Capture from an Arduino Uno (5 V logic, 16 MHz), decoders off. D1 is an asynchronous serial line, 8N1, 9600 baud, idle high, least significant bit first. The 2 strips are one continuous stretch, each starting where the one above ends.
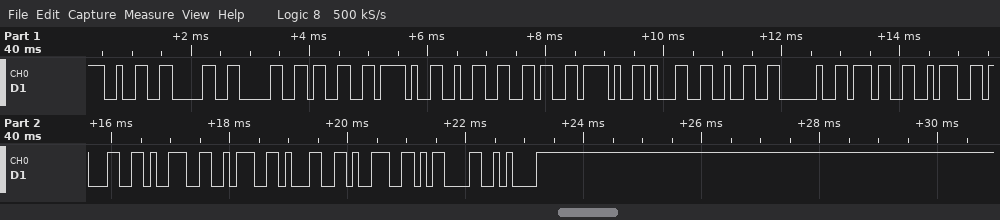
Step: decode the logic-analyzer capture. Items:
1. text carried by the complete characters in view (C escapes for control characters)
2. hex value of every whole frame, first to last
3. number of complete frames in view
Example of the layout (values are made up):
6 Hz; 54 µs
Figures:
"2003/26/12 7:19:19\r\n"; 0x32 0x30 0x30 0x33 0x2F 0x32 0x36 0x2F 0x31 0x32 0x20 0x37 0x3A 0x31 0x39 0x3A 0x31 0x39 0x0D 0x0A; 20
